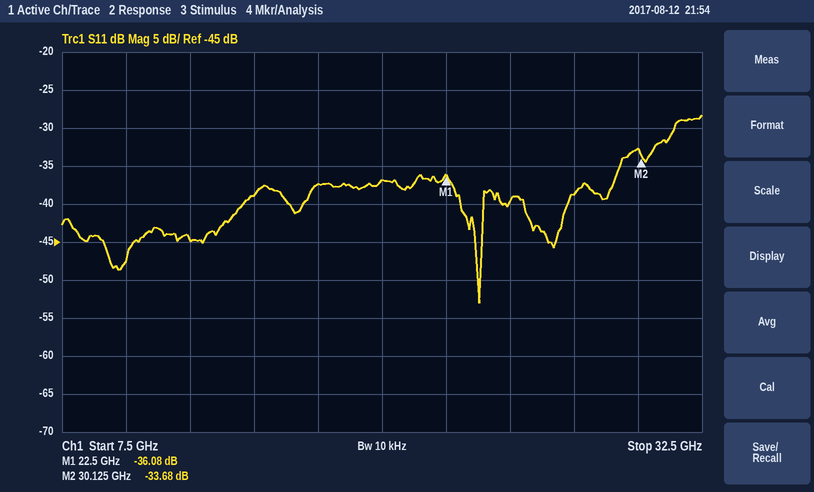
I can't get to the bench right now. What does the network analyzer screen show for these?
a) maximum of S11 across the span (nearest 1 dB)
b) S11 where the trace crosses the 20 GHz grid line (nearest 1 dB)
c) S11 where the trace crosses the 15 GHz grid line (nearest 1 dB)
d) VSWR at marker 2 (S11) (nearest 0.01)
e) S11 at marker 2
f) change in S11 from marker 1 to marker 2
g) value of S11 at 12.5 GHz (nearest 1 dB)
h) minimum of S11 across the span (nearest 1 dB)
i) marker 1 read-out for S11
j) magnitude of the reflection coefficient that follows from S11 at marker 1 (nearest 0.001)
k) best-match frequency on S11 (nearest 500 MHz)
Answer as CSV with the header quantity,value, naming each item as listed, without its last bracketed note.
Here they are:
quantity,value
maximum of S11 across the span,-28 dB
S11 where the trace crosses the 20 GHz grid line,-37 dB
S11 where the trace crosses the 15 GHz grid line,-39 dB
VSWR at marker 2 (S11),1.04
S11 at marker 2,-33.68 dB
change in S11 from marker 1 to marker 2,2.40 dB
value of S11 at 12.5 GHz,-45 dB
minimum of S11 across the span,-53 dB
marker 1 read-out for S11,-36.08 dB
magnitude of the reflection coefficient that follows from S11 at marker 1,0.016
best-match frequency on S11,24.0 GHz
